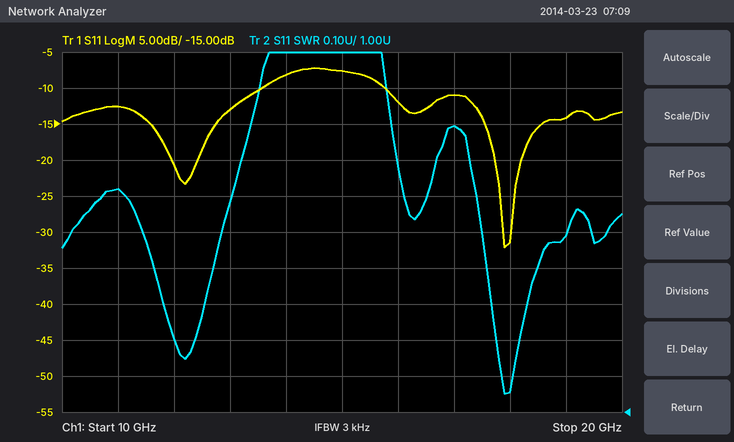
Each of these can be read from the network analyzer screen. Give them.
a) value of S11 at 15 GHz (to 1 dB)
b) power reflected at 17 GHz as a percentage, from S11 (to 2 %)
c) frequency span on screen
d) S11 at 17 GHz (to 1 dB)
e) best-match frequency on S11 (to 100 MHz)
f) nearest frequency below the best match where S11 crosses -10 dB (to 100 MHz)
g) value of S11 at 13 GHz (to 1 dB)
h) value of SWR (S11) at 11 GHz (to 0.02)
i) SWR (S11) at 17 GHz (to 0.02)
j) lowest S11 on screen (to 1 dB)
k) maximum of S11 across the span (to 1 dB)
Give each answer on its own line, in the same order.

-8 dB
8 %
10 GHz
-11 dB
17.9 GHz
15.8 GHz
-13 dB
1.62
1.80
-32 dB
-7 dB
